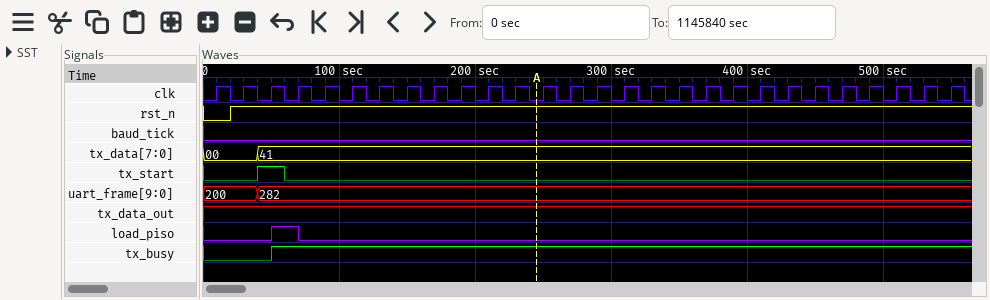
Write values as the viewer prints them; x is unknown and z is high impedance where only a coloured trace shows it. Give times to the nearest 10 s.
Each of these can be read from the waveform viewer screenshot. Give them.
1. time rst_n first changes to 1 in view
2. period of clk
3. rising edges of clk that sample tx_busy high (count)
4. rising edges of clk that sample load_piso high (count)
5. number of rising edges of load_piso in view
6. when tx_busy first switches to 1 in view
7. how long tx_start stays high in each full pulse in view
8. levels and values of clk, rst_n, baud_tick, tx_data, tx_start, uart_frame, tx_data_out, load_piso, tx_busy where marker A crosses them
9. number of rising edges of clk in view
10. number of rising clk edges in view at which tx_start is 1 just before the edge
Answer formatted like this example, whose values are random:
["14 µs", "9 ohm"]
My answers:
["20 s", "20 s", "25", "1", "1", "50 s", "20 s", "clk=0, rst_n=1, baud_tick=0, tx_data=41, tx_start=0, uart_frame=282, tx_data_out=1, load_piso=0, tx_busy=1", "28", "1"]
